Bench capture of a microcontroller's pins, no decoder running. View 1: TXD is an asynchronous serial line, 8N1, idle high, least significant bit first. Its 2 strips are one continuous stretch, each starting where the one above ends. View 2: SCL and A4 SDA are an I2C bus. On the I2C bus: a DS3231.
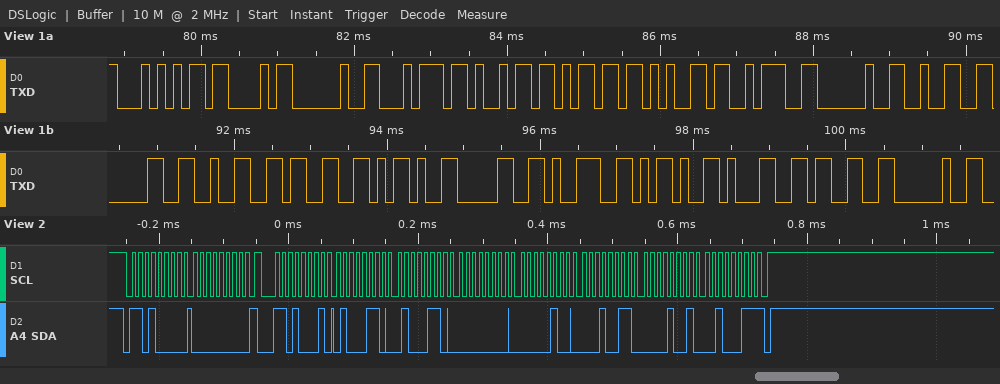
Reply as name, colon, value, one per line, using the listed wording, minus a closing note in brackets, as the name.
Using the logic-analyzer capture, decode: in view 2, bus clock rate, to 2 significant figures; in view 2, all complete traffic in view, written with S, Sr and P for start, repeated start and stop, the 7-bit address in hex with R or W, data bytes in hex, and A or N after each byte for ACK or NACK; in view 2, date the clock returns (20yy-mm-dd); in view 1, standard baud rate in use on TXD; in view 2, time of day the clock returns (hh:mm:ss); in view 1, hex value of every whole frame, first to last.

in view 2, bus clock rate, to 2 significant figures: 100 kHz
in view 2, all complete traffic in view, written with S, Sr and P for start, repeated start and stop, the 7-bit address in hex with R or W, data bytes in hex, and A or N after each byte for ACK or NACK: S 68W A 00 A Sr 68R A 46 A 46 A 00 A 04 A 13 A 09 A 23 N P
in view 2, date the clock returns: 2023-09-13
in view 1, standard baud rate in use on TXD: 9600 baud
in view 2, time of day the clock returns: 00:46:46
in view 1, hex value of every whole frame, first to last: 54 43 20 74 69 6D 65 3A 20 32 30 32 33 2D 30 39 2D 31 33 20
